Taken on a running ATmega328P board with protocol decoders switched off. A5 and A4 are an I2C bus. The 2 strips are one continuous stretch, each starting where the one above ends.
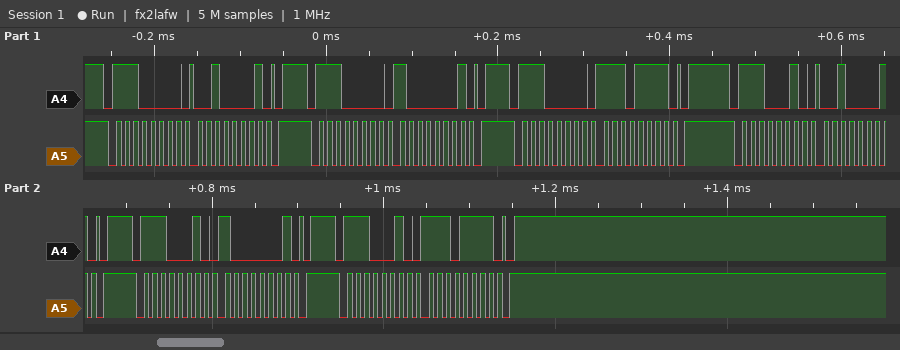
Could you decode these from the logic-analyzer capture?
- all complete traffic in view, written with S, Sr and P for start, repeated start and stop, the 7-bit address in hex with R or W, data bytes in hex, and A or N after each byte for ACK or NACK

S 70W A 21 A P S 70W A 81 A P S 70W A EF A P S 71W A 21 A P S 71W A 81 A P S 71W A EF A P
